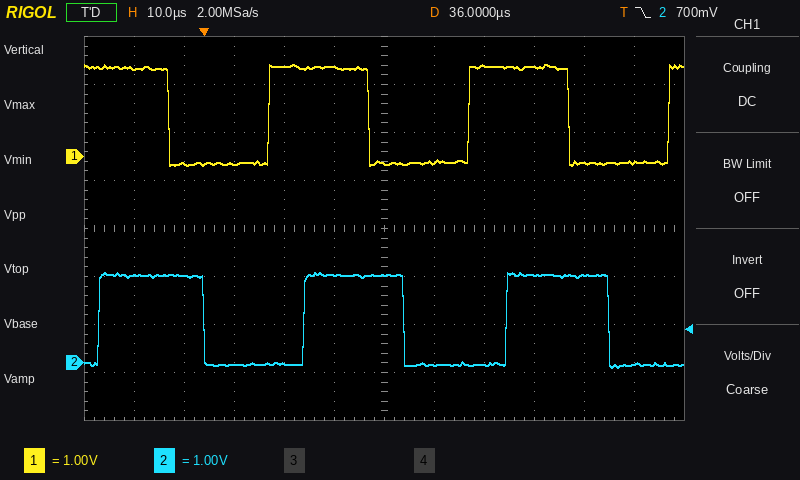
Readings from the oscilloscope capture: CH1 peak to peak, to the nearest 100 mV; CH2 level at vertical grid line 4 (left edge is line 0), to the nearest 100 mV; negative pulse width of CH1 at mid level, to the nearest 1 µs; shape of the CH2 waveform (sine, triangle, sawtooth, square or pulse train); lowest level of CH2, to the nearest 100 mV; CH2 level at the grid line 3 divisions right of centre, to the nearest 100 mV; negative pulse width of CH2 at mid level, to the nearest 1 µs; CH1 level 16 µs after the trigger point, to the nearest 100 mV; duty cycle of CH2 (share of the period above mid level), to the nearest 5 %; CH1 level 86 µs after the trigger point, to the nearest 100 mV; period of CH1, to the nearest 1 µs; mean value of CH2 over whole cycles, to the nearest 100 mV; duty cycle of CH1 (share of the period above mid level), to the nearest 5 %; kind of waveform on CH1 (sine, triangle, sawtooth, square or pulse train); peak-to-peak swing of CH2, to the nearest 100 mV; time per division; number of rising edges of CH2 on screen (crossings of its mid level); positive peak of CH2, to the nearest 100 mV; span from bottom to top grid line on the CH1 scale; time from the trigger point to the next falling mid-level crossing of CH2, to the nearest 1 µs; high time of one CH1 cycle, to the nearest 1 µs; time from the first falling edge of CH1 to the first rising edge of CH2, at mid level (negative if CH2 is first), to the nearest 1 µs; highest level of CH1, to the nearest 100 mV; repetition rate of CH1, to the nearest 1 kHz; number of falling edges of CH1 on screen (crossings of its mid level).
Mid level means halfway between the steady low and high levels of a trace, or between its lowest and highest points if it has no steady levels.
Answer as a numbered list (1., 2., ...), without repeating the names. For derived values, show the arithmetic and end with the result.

1. 1.9 V − (-200 mV) = 2.1 V
2. 0.0 V
3. 20 µs
4. square
5. -100 mV
6. 1.8 V
7. 20 µs
8. 1.9 V
9. 50 %
10. -100 mV
11. 40 µs
12. -100 mV + 0.5 × (1.9 V − (-100 mV)) ≈ 900 mV
13. 20 µs / 40 µs ≈ 50 %
14. square
15. 1.9 V − (-100 mV) = 2.0 V
16. 10 µs
17. 3
18. 1.9 V
19. 8 V
20. 40 µs
21. 20 µs
22. -14 µs
23. 1.9 V
24. 1 / 40 µs ≈ 25 kHz
25. 3
